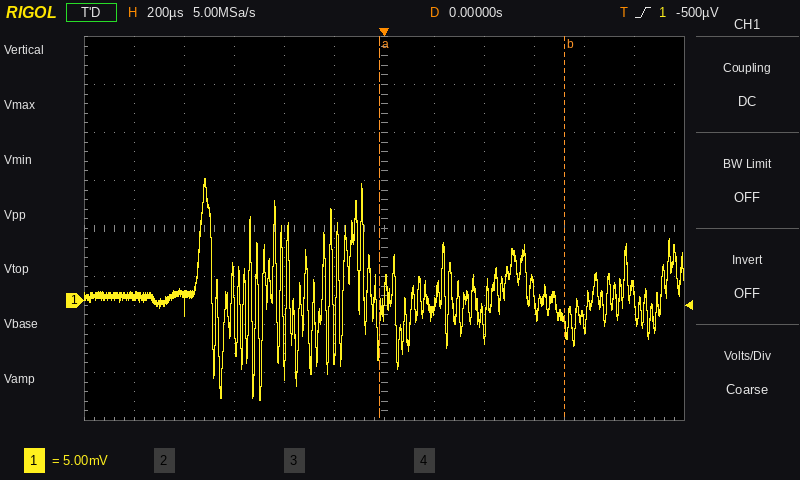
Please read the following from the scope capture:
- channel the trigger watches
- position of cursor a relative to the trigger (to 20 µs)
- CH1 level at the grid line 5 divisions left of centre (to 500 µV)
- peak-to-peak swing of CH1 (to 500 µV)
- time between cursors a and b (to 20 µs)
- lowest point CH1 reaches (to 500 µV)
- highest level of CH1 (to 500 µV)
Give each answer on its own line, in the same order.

CH1
-20 µs
500 µV
23.0 mV
740 µs
-10.5 mV
12.5 mV
